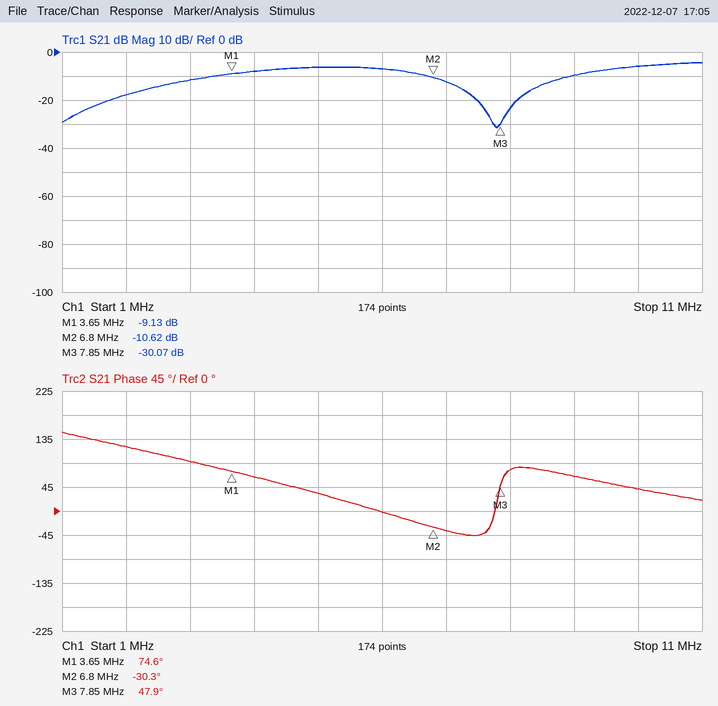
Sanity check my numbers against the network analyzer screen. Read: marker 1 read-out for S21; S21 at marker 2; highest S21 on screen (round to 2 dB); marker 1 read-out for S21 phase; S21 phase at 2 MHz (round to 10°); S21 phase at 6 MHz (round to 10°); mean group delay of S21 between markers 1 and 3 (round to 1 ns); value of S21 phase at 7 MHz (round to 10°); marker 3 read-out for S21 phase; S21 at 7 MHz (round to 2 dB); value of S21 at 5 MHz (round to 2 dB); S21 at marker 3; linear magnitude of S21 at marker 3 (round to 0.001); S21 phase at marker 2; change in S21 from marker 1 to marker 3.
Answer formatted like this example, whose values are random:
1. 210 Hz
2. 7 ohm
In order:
1. -9.13 dB
2. -10.62 dB
3. -4 dB
4. 74.6°
5. 120°
6. 0°
7. 18 ns
8. -40°
9. 47.9°
10. -12 dB
11. -6 dB
12. -30.07 dB
13. 0.031
14. -30.3°
15. -20.94 dB
